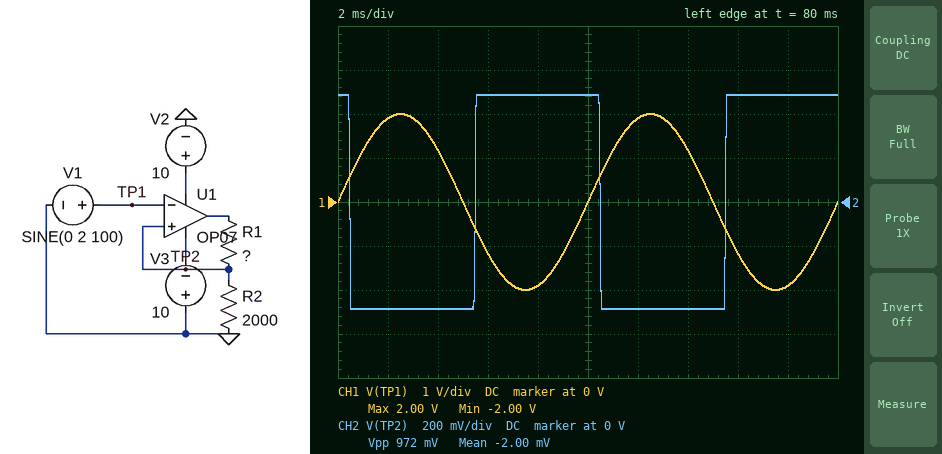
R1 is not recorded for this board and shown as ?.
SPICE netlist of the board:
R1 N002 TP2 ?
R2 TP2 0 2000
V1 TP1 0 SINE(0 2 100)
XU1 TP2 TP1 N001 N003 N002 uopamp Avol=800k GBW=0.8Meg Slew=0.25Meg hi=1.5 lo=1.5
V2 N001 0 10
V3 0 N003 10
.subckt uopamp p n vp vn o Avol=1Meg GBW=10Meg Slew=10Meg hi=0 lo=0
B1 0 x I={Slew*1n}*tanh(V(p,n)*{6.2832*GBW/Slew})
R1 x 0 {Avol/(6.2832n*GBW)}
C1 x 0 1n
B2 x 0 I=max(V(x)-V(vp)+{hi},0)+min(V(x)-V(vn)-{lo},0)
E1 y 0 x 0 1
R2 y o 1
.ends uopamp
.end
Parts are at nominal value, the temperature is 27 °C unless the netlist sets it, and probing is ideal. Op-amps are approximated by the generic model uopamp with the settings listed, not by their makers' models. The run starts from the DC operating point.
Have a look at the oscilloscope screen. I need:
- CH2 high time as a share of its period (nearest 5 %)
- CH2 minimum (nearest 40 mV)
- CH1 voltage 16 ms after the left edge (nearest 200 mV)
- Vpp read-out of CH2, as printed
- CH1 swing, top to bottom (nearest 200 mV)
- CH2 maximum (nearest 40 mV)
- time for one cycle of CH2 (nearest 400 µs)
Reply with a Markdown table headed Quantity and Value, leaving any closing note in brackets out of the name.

| Quantity | Value |
|---|---|
| CH2 high time as a share of its period | 50 % |
| CH2 minimum | -480 mV |
| CH1 voltage 16 ms after the left edge | -1.2 V |
| Vpp read-out of CH2, as printed | 972 mV |
| CH1 swing, top to bottom | 4.0 V |
| CH2 maximum | 480 mV |
| time for one cycle of CH2 | 10.0 ms |
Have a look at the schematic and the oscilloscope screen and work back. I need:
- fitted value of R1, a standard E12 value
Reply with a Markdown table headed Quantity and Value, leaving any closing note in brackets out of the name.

| Quantity | Value |
|---|---|
| fitted value of R1, a standard E12 value | 33 kΩ |
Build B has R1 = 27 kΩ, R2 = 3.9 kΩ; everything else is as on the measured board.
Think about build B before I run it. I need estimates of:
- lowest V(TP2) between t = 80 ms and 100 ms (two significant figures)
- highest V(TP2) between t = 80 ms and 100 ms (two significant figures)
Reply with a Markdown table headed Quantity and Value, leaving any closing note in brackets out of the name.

| Quantity | Value |
|---|---|
| lowest V(TP2) between t = 80 ms and 100 ms | -1.1 V |
| highest V(TP2) between t = 80 ms and 100 ms | 1.1 V |
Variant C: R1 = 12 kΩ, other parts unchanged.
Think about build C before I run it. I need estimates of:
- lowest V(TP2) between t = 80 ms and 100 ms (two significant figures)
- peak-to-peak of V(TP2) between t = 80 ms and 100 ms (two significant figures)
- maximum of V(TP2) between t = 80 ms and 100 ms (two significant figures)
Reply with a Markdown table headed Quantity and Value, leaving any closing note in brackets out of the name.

| Quantity | Value |
|---|---|
| lowest V(TP2) between t = 80 ms and 100 ms | -1.2 V |
| peak-to-peak of V(TP2) between t = 80 ms and 100 ms | 2.4 V |
| maximum of V(TP2) between t = 80 ms and 100 ms | 1.2 V |
